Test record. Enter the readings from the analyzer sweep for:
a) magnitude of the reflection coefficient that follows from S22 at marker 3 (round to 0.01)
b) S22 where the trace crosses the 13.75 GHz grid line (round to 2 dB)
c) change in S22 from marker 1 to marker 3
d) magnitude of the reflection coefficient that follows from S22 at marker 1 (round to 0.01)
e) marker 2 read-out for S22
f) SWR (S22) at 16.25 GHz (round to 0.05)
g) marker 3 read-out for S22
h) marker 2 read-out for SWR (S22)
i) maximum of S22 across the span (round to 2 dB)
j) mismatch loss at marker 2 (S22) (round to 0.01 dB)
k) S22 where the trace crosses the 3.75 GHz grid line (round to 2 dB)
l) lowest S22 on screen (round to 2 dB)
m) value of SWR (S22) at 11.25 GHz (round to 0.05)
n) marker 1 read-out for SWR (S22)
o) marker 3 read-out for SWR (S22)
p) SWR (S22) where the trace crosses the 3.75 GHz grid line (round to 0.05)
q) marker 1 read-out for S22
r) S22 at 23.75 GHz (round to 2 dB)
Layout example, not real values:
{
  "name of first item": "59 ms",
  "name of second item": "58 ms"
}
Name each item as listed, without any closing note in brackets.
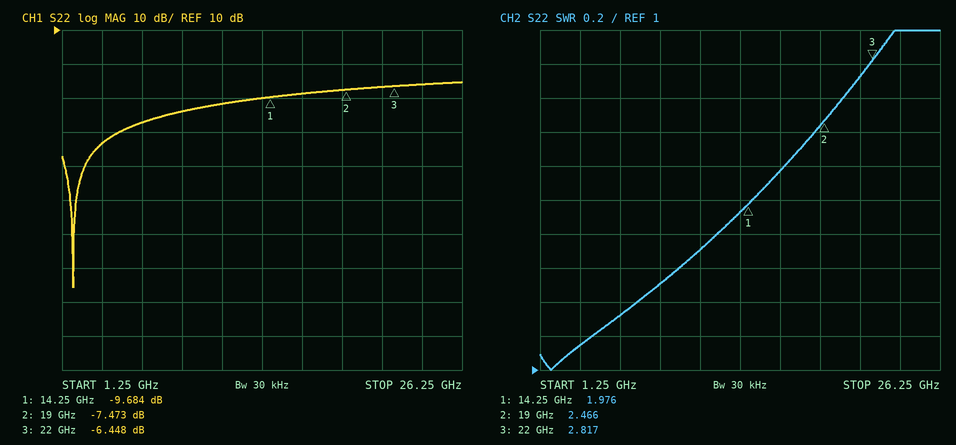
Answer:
{
  "magnitude of the reflection coefficient that follows from S22 at marker 3": "0.48",
  "S22 where the trace crosses the 13.75 GHz grid line": "-10 dB",
  "change in S22 from marker 1 to marker 3": "3.236 dB",
  "magnitude of the reflection coefficient that follows from S22 at marker 1": "0.33",
  "marker 2 read-out for S22": "-7.473 dB",
  "SWR (S22) at 16.25 GHz": "2.15",
  "marker 3 read-out for S22": "-6.448 dB",
  "marker 2 read-out for SWR": "2.466",
  "maximum of S22 across the span": "-6 dB",
  "mismatch loss at marker 2 (S22)": "0.86 dB",
  "S22 where the trace crosses the 3.75 GHz grid line": "-24 dB",
  "lowest S22 on screen": "-66 dB",
  "value of SWR (S22) at 11.25 GHz": "1.70",
  "marker 1 read-out for SWR": "1.976",
  "marker 3 read-out for SWR": "2.817",
  "SWR (S22) where the trace crosses the 3.75 GHz grid line": "1.15",
  "marker 1 read-out for S22": "-9.684 dB",
  "S22 at 23.75 GHz": "-6 dB"
}
